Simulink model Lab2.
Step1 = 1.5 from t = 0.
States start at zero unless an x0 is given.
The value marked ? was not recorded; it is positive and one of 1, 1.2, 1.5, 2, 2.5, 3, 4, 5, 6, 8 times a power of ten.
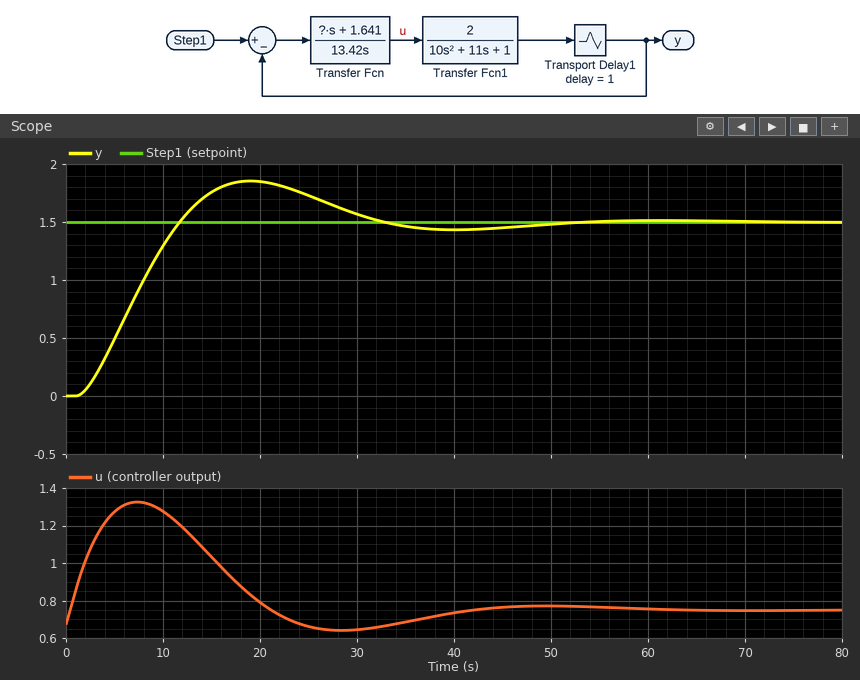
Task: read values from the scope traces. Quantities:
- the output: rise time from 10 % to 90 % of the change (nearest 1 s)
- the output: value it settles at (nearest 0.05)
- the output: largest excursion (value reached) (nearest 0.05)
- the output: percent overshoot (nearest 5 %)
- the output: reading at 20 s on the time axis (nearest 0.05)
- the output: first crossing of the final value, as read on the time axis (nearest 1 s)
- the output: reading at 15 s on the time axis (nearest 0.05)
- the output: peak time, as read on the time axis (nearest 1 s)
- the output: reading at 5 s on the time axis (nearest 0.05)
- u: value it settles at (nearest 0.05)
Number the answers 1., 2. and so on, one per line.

1. 8 s
2. 1.50
3. 1.85
4. 25 %
5. 1.85
6. 12 s
7. 1.75
8. 19 s
9. 0.50
10. 0.75
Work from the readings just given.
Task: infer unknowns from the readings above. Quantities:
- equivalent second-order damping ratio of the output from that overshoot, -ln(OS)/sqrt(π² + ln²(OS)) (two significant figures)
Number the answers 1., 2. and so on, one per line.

1. 0.40
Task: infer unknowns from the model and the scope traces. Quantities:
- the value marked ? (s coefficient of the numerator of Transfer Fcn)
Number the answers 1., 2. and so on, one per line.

1. 6
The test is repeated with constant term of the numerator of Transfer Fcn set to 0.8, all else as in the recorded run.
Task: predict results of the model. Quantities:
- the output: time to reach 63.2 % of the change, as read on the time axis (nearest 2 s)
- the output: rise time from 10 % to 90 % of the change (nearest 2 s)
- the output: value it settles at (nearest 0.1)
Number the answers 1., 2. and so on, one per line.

1. 10 s
2. 14 s
3. 1.5
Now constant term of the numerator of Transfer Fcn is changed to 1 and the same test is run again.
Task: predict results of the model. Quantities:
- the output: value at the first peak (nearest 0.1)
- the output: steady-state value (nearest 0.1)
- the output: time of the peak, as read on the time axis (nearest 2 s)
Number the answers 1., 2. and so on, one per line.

1. 1.6
2. 1.5
3. 26 s
